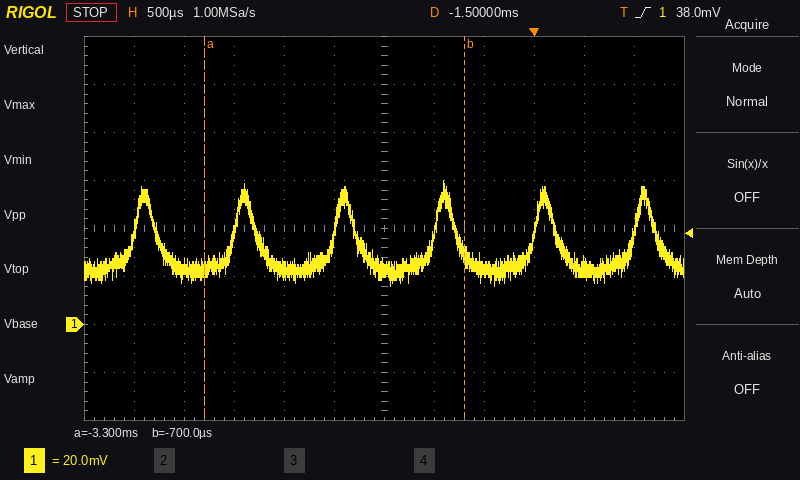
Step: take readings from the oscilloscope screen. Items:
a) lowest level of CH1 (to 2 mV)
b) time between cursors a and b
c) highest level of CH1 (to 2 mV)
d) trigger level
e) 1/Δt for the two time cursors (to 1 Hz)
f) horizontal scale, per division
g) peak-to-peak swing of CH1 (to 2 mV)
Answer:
16 mV
2.60 ms
60 mV
38.0 mV
385 Hz
500 µs
44 mV
